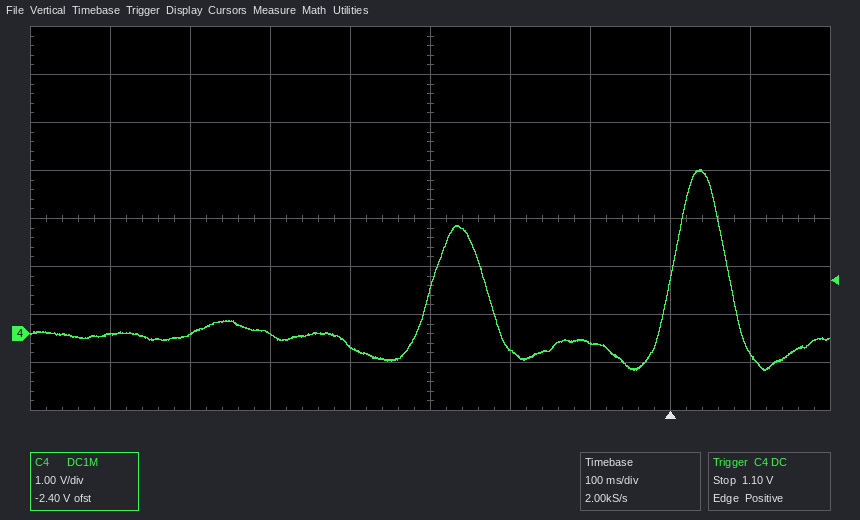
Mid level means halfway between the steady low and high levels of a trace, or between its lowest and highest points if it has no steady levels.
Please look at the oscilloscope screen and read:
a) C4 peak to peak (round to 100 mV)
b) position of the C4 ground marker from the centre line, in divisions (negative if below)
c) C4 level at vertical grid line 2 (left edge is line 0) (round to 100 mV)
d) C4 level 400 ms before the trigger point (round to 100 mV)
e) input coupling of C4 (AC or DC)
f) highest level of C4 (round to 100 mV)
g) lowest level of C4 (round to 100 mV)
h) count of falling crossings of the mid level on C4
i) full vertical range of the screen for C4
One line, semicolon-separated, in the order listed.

4.2 V; -2.4 div; 0.0 V; -300 mV; DC; 3.4 V; -800 mV; 2; 8 V
